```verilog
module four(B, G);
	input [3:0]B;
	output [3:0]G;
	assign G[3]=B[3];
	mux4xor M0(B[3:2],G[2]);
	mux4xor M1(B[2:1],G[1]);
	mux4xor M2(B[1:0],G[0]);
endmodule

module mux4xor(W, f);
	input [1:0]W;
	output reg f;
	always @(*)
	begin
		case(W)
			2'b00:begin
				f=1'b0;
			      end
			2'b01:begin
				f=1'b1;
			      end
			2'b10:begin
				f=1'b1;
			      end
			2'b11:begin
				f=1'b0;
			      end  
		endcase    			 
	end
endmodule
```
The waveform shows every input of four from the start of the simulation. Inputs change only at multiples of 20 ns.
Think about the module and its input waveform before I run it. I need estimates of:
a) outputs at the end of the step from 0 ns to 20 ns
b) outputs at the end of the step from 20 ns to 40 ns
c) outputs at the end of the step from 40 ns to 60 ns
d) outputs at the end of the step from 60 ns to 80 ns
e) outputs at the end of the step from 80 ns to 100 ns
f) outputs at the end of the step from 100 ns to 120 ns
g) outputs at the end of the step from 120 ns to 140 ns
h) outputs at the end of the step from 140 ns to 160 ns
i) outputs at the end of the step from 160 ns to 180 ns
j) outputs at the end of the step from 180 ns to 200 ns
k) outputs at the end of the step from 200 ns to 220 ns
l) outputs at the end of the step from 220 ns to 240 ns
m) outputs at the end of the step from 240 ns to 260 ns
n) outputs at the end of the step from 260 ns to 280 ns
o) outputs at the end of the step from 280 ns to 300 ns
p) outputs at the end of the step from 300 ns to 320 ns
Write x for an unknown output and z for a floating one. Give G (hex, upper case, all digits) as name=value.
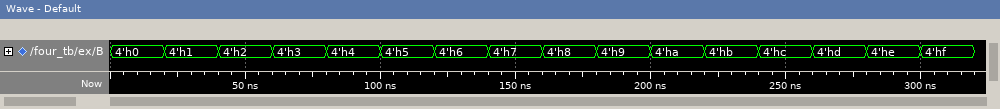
G=0
G=1
G=3
G=2
G=6
G=7
G=5
G=4
G=C
G=D
G=F
G=E
G=A
G=B
G=9
G=8
